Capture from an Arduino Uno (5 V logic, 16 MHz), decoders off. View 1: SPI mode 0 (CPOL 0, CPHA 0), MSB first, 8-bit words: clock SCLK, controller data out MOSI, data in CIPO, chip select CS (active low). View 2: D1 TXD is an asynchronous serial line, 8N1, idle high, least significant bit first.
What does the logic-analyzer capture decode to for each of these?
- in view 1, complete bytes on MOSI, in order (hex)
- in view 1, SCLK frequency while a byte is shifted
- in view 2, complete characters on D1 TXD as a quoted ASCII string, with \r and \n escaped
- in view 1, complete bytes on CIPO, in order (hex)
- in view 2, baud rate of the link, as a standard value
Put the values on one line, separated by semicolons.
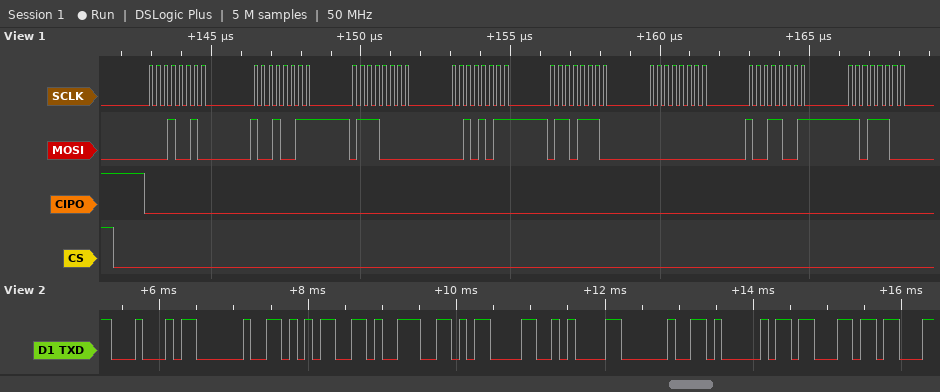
0x12 0x93 0x70 0x2B 0x6E 0x00 0x99 0xDC; 4 MHz; "D 59\r\n Ac"; 0x00 0x00 0x00 0x00 0x00 0x00 0x00 0x00; 9600 baud
